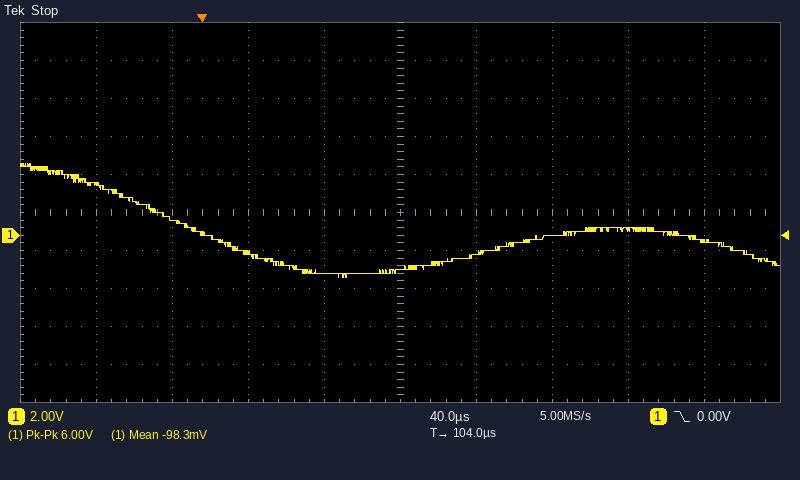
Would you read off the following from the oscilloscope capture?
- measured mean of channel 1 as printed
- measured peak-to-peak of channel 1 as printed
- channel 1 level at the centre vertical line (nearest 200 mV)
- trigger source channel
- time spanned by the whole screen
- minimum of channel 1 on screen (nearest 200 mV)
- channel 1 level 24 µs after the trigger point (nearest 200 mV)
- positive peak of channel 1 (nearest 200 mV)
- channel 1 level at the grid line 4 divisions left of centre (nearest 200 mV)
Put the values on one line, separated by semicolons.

-98.3 mV; 6.00 V; -1.8 V; channel 1; 400 µs; -2.2 V; -1.0 V; 3.8 V; 2.6 V
